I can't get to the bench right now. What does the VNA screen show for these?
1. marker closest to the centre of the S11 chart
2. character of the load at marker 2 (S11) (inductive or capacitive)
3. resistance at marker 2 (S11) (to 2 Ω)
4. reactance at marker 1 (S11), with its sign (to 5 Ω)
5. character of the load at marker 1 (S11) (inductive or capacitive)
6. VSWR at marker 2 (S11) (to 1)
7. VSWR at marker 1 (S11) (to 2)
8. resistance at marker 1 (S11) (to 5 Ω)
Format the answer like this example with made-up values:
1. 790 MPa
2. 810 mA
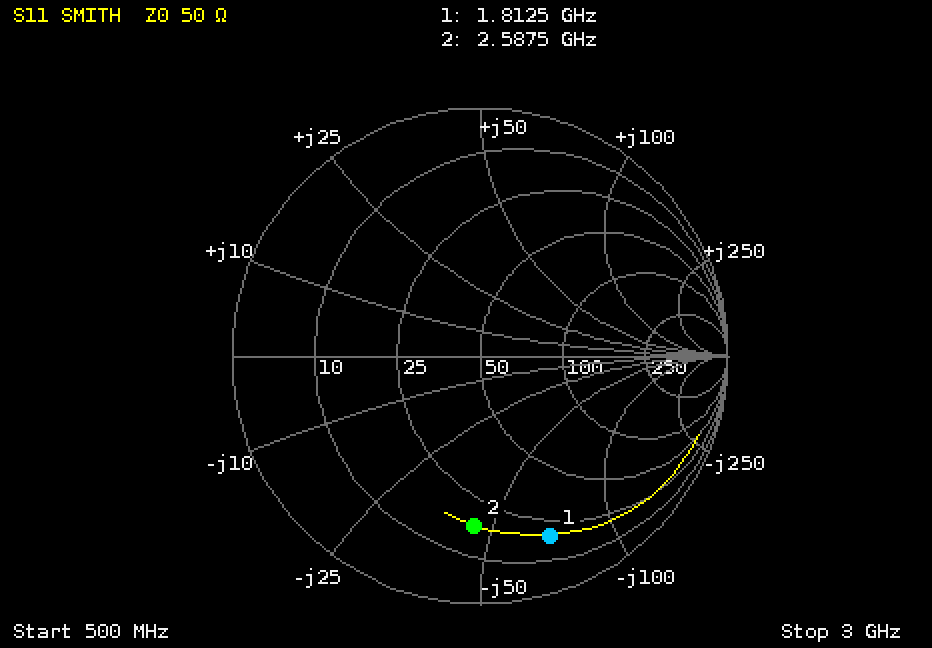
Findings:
1. marker 2
2. capacitive
3. 18 Ω
4. -70 Ω
5. capacitive
6. 5
7. 8
8. 20 Ω
